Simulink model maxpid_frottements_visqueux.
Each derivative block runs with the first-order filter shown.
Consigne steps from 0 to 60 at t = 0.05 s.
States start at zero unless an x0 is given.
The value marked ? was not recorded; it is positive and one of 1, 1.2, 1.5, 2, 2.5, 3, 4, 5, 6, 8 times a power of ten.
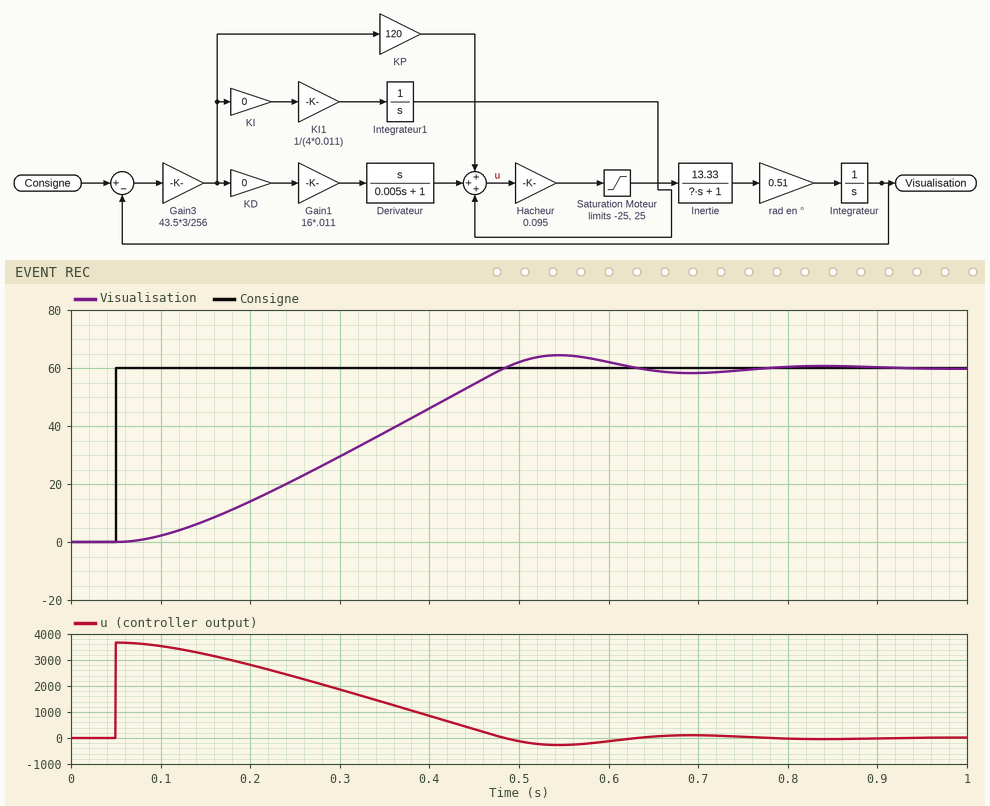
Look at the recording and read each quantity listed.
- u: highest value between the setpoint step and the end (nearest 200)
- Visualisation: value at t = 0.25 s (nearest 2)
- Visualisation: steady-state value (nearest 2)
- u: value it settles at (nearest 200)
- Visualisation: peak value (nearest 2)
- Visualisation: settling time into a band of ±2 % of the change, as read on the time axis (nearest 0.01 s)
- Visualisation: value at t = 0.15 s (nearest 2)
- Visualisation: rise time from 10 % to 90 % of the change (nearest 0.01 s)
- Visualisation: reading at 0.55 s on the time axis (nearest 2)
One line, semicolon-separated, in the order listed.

3600; 22; 60; 0; 64; 0.73 s; 8; 0.31 s; 64
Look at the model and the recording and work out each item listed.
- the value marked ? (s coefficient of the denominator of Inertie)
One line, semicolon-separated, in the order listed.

0.08
